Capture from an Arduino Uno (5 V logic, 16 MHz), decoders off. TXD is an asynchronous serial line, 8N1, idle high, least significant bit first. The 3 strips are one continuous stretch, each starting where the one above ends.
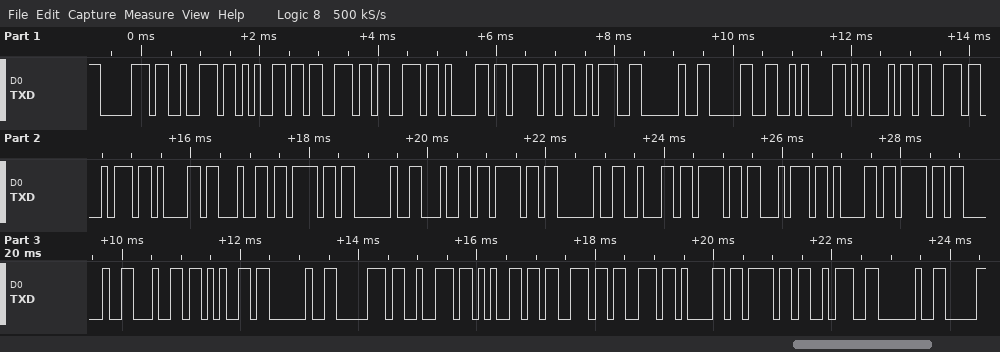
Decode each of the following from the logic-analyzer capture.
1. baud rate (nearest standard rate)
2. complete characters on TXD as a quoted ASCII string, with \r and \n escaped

9600 baud
"pressao: 0\nEstado do botao de pressao: "
